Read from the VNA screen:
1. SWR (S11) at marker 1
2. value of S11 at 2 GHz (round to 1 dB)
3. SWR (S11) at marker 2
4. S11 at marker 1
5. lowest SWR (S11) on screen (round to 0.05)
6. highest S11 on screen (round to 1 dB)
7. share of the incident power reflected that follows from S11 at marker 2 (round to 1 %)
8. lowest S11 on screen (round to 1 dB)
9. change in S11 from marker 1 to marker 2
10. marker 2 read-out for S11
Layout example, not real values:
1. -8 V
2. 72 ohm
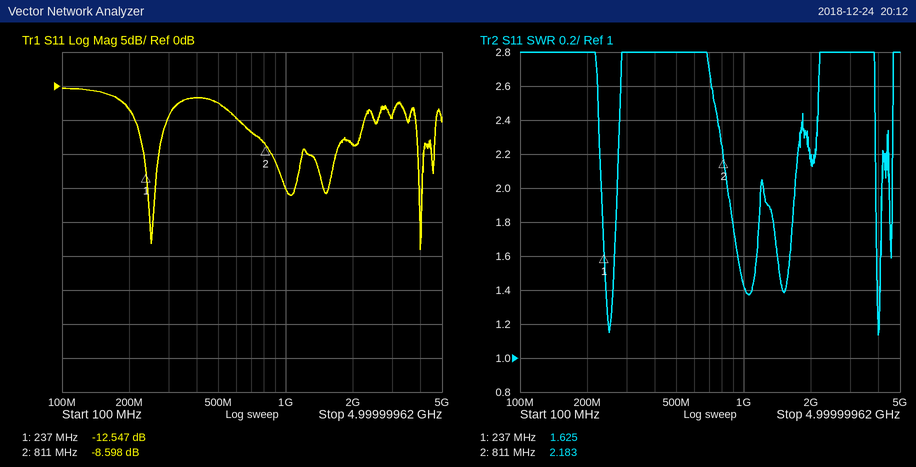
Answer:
1. 1.625
2. -9 dB
3. 2.183
4. -12.547 dB
5. 1.15
6. 0 dB
7. 14 %
8. -24 dB
9. 3.949 dB
10. -8.598 dB
